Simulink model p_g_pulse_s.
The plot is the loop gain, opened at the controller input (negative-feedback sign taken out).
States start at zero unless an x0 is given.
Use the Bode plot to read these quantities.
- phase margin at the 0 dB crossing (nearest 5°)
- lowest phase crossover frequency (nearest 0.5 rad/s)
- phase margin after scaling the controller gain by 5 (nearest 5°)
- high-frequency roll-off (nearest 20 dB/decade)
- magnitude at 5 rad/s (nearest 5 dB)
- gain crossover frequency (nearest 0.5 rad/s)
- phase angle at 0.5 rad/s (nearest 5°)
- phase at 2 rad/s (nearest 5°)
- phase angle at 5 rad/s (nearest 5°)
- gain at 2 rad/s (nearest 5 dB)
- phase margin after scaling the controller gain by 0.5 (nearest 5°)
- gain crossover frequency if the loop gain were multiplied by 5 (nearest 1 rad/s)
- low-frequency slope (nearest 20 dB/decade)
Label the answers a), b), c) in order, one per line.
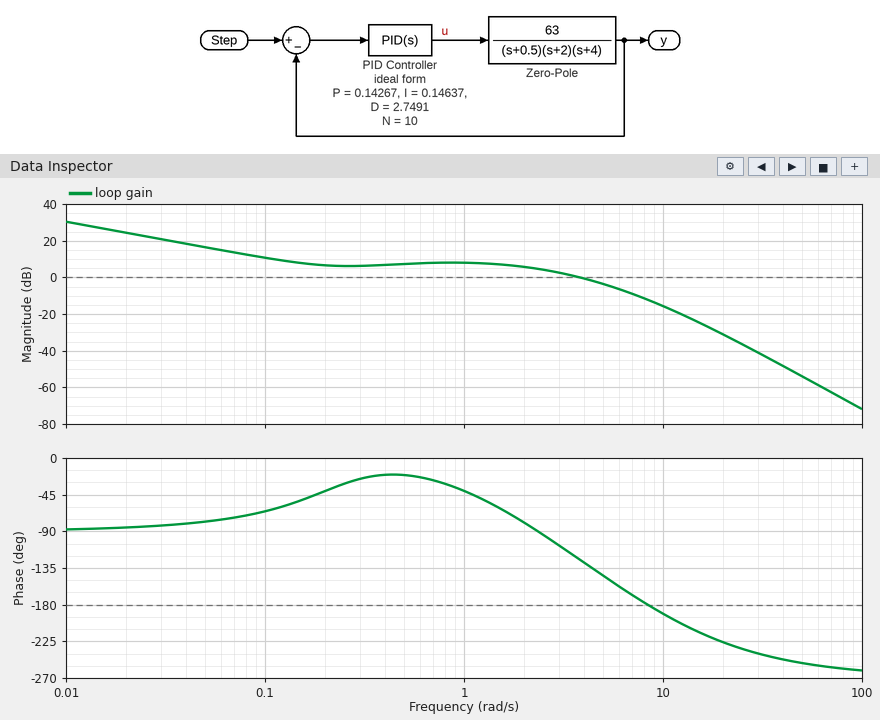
a) 55°
b) 8.5 rad/s
c) -5°
d) -60 dB/decade
e) -5 dB
f) 4.0 rad/s
g) -20°
h) -80°
i) -145°
j) 5 dB
k) 105°
l) 9 rad/s
m) -20 dB/decade
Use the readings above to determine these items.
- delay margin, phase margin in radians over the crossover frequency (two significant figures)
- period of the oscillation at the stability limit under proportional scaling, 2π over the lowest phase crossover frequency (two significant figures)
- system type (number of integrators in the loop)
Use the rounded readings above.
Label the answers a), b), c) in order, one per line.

a) 0.24 s
b) 0.74 s
c) 1
